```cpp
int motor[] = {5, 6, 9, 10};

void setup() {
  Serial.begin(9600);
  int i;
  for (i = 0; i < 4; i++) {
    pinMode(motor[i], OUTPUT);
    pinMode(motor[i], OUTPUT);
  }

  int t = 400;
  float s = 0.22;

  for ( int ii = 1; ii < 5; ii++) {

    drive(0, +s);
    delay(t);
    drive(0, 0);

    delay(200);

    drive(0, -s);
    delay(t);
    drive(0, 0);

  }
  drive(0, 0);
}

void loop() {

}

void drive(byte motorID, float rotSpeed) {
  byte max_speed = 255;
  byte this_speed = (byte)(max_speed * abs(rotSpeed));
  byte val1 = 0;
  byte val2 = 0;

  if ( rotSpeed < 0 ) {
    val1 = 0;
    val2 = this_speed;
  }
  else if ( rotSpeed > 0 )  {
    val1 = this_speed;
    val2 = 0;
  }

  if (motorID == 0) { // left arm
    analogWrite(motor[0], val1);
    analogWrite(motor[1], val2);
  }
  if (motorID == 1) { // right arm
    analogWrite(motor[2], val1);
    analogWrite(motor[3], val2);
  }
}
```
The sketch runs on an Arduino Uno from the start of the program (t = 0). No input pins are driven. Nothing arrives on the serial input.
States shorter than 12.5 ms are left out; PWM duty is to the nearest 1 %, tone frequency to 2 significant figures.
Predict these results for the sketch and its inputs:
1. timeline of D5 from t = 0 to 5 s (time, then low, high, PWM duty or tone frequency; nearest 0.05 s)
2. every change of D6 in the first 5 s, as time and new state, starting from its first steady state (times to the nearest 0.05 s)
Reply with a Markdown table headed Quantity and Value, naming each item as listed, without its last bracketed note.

| Quantity | Value |
|---|---|
| timeline of D5 from t = 0 to 5 s | 0 s PWM 22 %; 0.4 s low; 1 s PWM 22 %; 1.4 s low; 2 s PWM 22 %; 2.4 s low; 3 s PWM 22 %; 3.4 s low |
| every change of D6 in the first 5 s, as time and new state, starting from its first steady state | 0 s low; 0.6 s PWM 22 %; 1 s low; 1.6 s PWM 22 %; 2 s low; 2.6 s PWM 22 %; 3 s low; 3.6 s PWM 22 %; 4 s low |
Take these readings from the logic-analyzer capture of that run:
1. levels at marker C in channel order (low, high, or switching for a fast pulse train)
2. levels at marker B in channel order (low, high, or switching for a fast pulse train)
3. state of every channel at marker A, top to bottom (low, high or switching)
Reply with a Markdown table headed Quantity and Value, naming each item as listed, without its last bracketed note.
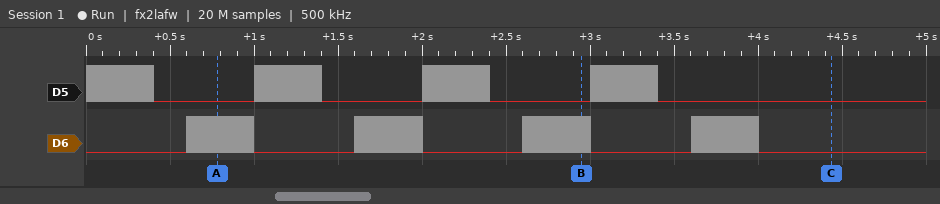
| Quantity | Value |
|---|---|
| levels at marker C in channel order | D5 low, D6 low |
| levels at marker B in channel order | D5 low, D6 switching |
| state of every channel at marker A, top to bottom | D5 low, D6 switching |
